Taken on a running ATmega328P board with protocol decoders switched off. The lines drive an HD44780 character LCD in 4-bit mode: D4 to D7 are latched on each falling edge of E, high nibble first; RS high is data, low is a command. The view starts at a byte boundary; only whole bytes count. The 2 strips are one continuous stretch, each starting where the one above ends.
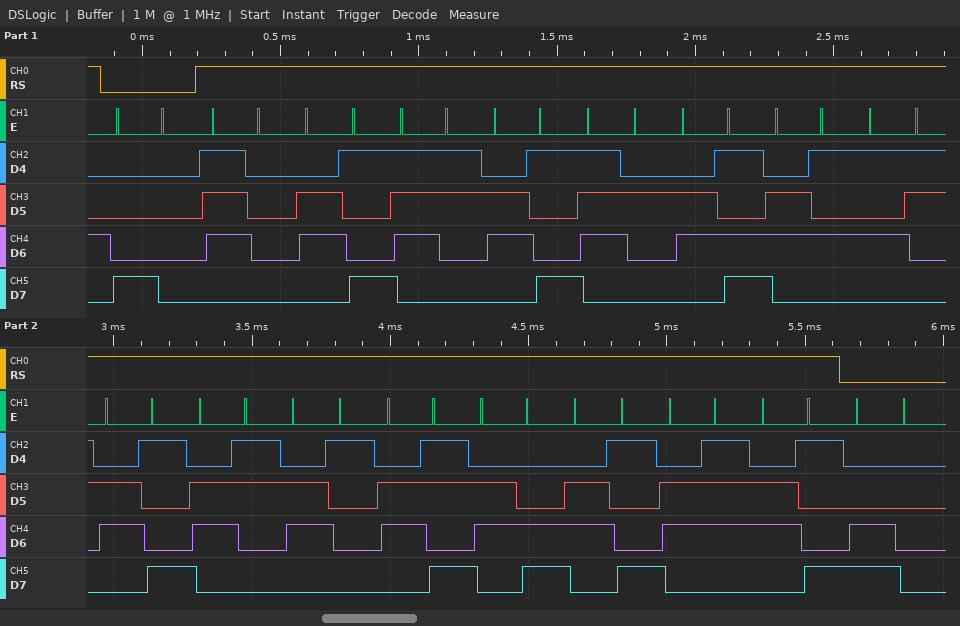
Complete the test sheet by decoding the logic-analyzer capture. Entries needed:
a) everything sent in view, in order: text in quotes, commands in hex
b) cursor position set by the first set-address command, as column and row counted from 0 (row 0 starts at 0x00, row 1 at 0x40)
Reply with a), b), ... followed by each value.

a) 0x80 "pisirmeSicakligi" 0xC0
b) column 0, row 0
